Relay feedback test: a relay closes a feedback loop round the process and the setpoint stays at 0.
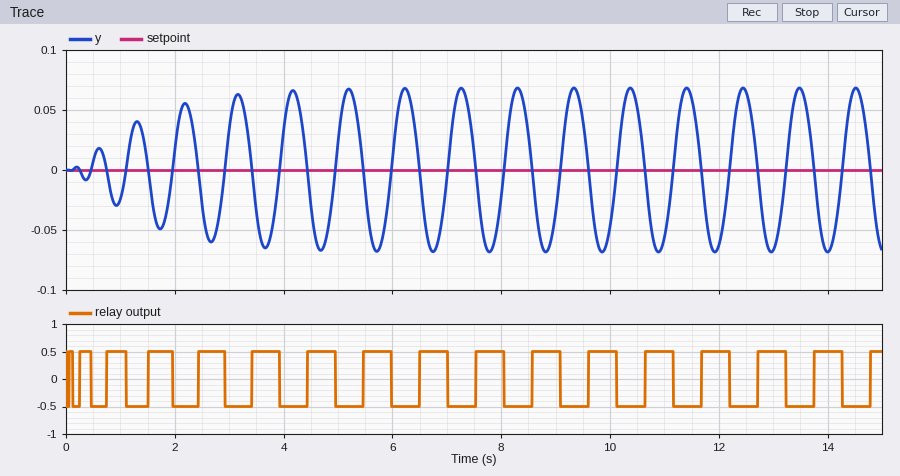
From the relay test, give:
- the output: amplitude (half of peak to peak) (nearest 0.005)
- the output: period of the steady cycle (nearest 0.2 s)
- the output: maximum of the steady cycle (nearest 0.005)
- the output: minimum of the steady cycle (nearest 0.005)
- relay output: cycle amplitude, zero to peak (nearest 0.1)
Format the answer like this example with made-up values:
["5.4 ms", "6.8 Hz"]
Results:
["0.070", "1.0 s", "0.070", "-0.070", "0.5"]
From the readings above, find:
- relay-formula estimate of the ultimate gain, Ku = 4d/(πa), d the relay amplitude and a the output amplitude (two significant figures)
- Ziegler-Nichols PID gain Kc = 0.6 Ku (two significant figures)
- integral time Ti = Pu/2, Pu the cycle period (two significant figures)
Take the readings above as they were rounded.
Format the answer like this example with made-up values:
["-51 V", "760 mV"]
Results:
["9.1", "5.5", "0.50 s"]
